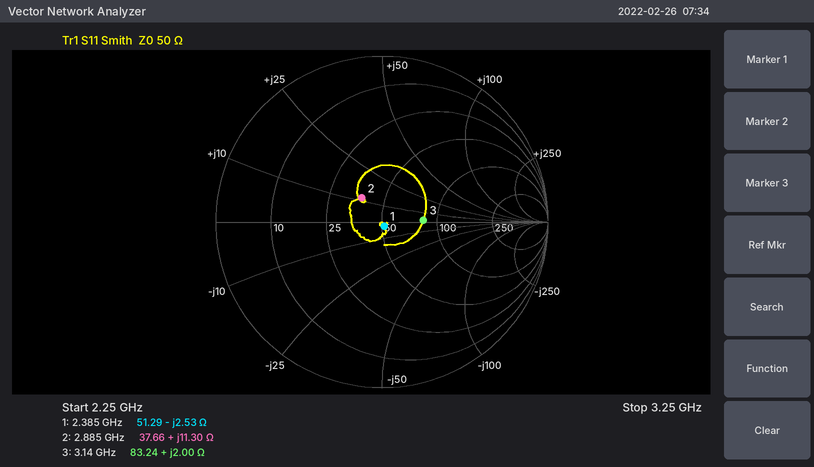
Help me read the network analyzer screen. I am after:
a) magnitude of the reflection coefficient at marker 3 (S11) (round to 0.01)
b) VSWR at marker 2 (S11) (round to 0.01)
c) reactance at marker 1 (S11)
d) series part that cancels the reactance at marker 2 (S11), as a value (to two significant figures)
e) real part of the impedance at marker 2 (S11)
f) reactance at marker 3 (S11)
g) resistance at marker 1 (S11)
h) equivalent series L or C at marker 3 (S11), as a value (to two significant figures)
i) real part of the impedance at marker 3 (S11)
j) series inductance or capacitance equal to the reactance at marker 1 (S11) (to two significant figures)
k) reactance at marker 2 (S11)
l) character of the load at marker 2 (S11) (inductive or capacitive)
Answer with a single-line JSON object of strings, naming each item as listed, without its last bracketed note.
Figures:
{"magnitude of the reflection coefficient at marker 3 (S11)": "0.25", "VSWR at marker 2 (S11)": "1.47", "reactance at marker 1": "-2.53 Ω", "series part that cancels the reactance at marker 2 (S11), as a value": "4.9 pF", "real part of the impedance at marker 2": "37.66 Ω", "reactance at marker 3": "+2.00 Ω", "resistance at marker 1": "51.29 Ω", "equivalent series L or C at marker 3 (S11), as a value": "100 pH", "real part of the impedance at marker 3": "83.24 Ω", "series inductance or capacitance equal to the reactance at marker 1 (S11)": "26 pF", "reactance at marker 2": "+11.30 Ω", "character of the load at marker 2 (S11)": "inductive"}
